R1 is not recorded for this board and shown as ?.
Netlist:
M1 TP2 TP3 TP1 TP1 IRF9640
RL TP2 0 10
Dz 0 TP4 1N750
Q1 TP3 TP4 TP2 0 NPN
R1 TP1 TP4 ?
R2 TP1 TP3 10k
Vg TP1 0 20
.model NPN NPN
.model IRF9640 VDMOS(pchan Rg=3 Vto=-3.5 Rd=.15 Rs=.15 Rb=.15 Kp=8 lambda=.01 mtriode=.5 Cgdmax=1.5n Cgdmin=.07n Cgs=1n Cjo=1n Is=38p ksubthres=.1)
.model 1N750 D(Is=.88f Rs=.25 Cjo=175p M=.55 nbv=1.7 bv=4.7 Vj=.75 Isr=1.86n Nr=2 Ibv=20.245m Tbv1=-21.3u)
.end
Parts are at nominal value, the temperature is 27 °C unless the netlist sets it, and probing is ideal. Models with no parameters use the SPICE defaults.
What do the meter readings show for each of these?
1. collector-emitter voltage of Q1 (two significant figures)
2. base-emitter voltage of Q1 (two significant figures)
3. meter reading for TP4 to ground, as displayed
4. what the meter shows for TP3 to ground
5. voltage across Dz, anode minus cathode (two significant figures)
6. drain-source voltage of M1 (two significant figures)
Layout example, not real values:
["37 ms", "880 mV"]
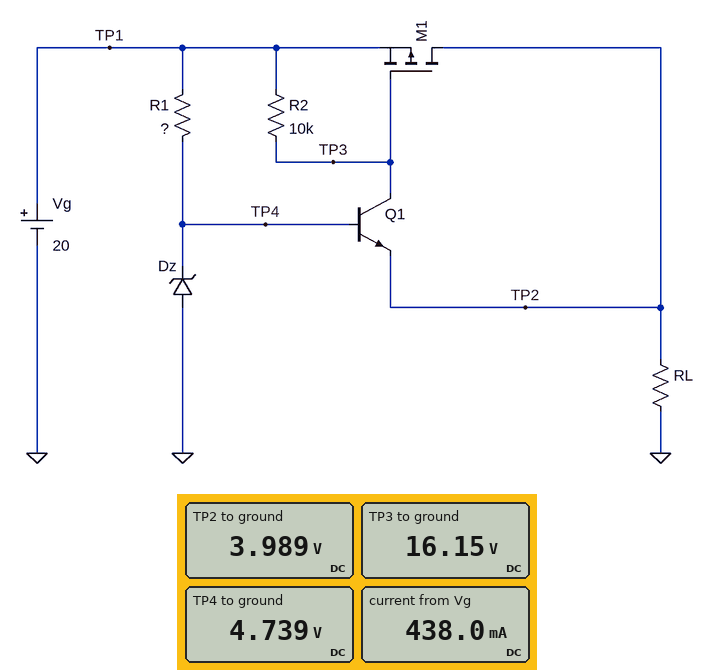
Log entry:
["12 V", "750 mV", "4.739 V", "16.15 V", "-4.7 V", "-16 V"]
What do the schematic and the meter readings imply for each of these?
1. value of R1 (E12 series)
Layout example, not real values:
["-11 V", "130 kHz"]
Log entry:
["390 Ω"]
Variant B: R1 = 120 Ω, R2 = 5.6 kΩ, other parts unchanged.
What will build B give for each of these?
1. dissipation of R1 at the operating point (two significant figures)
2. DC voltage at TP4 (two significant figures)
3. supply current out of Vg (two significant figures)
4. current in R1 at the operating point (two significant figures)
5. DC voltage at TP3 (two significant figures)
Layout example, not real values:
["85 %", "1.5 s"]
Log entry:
["1.9 W", "4.8 V", "530 mA", "130 mA", "16 V"]
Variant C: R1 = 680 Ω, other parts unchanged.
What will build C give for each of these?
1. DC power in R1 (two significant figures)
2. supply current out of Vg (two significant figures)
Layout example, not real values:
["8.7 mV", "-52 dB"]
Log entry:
["340 mW", "420 mA"]
